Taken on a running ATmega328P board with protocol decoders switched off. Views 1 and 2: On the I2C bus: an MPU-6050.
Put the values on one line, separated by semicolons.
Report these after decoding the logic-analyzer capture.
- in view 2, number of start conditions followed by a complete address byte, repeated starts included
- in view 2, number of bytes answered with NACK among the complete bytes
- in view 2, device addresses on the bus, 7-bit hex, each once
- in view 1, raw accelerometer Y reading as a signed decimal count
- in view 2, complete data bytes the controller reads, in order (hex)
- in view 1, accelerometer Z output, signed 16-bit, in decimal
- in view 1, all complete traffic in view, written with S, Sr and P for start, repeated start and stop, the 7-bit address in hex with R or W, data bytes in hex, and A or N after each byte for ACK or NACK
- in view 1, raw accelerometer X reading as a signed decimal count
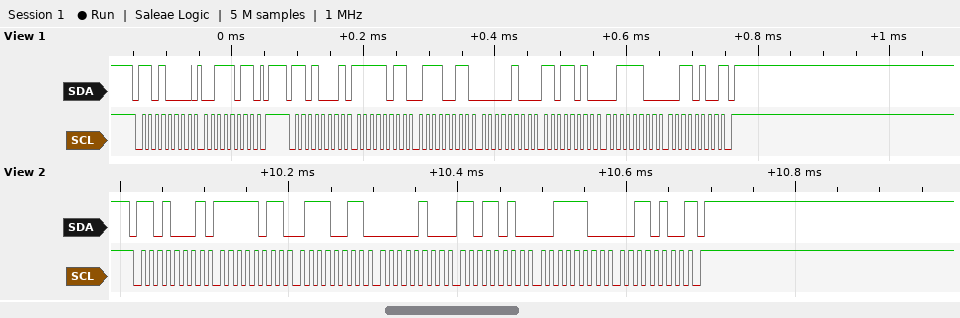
1; 1; 0x68; 1242; FB 73 04 DA 3C 34; 15412; S 68W A 3B A P S 68R A FB A 73 A 04 A DA A 3C A 34 N P; -1165
